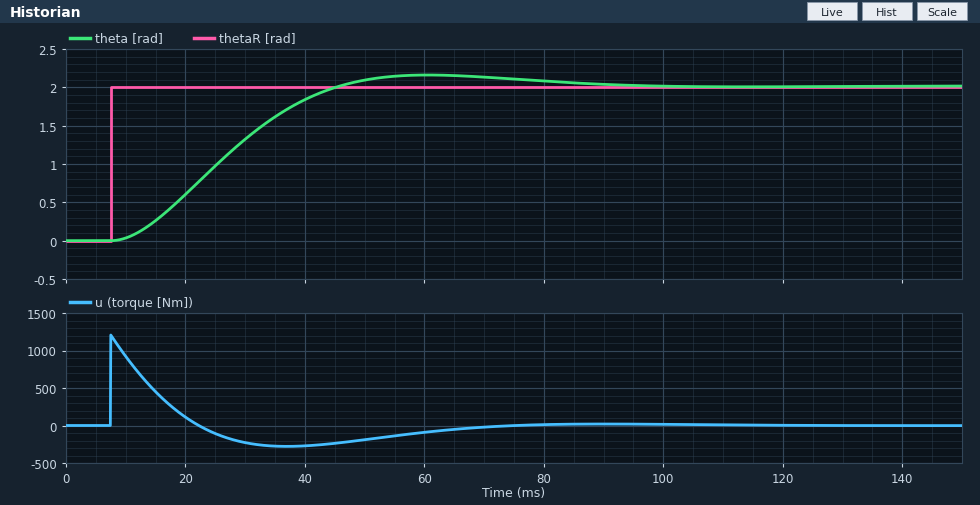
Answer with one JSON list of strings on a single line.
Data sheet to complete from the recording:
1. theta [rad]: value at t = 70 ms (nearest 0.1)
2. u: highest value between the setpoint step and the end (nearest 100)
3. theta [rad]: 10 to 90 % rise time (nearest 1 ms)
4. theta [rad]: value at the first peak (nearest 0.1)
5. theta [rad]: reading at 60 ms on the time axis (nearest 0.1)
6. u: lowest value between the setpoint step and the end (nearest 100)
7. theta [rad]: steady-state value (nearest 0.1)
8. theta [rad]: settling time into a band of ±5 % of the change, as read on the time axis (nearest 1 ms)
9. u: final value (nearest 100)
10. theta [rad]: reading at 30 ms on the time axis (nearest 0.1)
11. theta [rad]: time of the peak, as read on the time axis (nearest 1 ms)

["2.1", "1200", "25 ms", "2.2", "2.2", "-300", "2.0", "73 ms", "0", "1.3", "61 ms"]
